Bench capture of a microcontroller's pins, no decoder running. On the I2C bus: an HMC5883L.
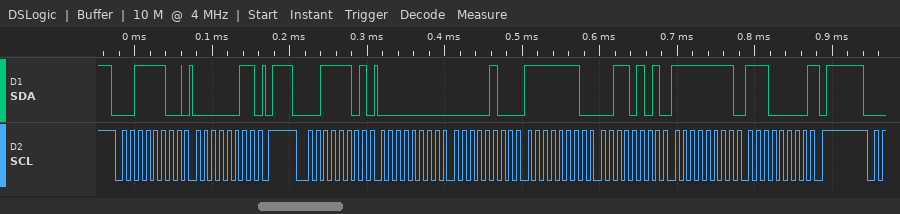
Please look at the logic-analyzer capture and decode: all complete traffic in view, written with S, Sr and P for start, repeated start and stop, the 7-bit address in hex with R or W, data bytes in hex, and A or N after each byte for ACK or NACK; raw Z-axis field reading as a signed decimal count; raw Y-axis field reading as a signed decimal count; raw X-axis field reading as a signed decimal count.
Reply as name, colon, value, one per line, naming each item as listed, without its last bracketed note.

all complete traffic in view, written with S, Sr and P for start, repeated start and stop, the 7-bit address in hex with R or W, data bytes in hex, and A or N after each byte for ACK or NACK: S 1EW A 03 A P S 1ER A 00 A 04 A FE A 35 A FF A E0 N P
raw Z-axis field reading as a signed decimal count: -459
raw Y-axis field reading as a signed decimal count: -32
raw X-axis field reading as a signed decimal count: 4
